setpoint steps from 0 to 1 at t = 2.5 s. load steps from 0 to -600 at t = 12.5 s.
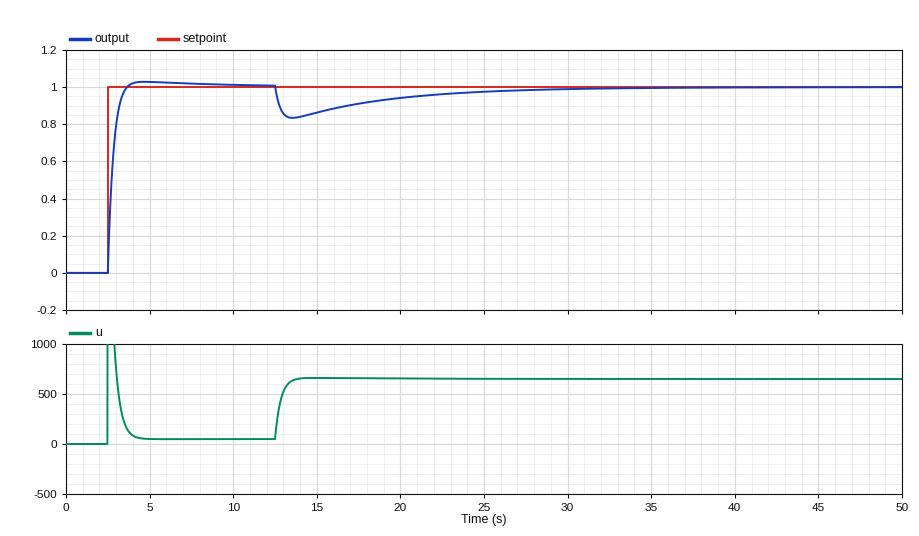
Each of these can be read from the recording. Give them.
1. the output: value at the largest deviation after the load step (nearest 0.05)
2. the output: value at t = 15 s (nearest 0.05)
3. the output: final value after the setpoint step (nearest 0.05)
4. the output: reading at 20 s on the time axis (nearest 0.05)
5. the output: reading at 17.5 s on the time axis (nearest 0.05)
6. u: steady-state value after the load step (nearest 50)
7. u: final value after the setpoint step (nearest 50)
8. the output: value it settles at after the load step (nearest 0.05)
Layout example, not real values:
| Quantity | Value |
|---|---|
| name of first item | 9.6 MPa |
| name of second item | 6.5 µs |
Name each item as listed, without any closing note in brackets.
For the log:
| Quantity | Value |
|---|---|
| the output: value at the largest deviation after the load step | 0.85 |
| the output: value at t = 15 s | 0.85 |
| the output: final value after the setpoint step | 1.00 |
| the output: reading at 20 s on the time axis | 0.95 |
| the output: reading at 17.5 s on the time axis | 0.90 |
| u: steady-state value after the load step | 650 |
| u: final value after the setpoint step | 50 |
| the output: value it settles at after the load step | 1.00 |
